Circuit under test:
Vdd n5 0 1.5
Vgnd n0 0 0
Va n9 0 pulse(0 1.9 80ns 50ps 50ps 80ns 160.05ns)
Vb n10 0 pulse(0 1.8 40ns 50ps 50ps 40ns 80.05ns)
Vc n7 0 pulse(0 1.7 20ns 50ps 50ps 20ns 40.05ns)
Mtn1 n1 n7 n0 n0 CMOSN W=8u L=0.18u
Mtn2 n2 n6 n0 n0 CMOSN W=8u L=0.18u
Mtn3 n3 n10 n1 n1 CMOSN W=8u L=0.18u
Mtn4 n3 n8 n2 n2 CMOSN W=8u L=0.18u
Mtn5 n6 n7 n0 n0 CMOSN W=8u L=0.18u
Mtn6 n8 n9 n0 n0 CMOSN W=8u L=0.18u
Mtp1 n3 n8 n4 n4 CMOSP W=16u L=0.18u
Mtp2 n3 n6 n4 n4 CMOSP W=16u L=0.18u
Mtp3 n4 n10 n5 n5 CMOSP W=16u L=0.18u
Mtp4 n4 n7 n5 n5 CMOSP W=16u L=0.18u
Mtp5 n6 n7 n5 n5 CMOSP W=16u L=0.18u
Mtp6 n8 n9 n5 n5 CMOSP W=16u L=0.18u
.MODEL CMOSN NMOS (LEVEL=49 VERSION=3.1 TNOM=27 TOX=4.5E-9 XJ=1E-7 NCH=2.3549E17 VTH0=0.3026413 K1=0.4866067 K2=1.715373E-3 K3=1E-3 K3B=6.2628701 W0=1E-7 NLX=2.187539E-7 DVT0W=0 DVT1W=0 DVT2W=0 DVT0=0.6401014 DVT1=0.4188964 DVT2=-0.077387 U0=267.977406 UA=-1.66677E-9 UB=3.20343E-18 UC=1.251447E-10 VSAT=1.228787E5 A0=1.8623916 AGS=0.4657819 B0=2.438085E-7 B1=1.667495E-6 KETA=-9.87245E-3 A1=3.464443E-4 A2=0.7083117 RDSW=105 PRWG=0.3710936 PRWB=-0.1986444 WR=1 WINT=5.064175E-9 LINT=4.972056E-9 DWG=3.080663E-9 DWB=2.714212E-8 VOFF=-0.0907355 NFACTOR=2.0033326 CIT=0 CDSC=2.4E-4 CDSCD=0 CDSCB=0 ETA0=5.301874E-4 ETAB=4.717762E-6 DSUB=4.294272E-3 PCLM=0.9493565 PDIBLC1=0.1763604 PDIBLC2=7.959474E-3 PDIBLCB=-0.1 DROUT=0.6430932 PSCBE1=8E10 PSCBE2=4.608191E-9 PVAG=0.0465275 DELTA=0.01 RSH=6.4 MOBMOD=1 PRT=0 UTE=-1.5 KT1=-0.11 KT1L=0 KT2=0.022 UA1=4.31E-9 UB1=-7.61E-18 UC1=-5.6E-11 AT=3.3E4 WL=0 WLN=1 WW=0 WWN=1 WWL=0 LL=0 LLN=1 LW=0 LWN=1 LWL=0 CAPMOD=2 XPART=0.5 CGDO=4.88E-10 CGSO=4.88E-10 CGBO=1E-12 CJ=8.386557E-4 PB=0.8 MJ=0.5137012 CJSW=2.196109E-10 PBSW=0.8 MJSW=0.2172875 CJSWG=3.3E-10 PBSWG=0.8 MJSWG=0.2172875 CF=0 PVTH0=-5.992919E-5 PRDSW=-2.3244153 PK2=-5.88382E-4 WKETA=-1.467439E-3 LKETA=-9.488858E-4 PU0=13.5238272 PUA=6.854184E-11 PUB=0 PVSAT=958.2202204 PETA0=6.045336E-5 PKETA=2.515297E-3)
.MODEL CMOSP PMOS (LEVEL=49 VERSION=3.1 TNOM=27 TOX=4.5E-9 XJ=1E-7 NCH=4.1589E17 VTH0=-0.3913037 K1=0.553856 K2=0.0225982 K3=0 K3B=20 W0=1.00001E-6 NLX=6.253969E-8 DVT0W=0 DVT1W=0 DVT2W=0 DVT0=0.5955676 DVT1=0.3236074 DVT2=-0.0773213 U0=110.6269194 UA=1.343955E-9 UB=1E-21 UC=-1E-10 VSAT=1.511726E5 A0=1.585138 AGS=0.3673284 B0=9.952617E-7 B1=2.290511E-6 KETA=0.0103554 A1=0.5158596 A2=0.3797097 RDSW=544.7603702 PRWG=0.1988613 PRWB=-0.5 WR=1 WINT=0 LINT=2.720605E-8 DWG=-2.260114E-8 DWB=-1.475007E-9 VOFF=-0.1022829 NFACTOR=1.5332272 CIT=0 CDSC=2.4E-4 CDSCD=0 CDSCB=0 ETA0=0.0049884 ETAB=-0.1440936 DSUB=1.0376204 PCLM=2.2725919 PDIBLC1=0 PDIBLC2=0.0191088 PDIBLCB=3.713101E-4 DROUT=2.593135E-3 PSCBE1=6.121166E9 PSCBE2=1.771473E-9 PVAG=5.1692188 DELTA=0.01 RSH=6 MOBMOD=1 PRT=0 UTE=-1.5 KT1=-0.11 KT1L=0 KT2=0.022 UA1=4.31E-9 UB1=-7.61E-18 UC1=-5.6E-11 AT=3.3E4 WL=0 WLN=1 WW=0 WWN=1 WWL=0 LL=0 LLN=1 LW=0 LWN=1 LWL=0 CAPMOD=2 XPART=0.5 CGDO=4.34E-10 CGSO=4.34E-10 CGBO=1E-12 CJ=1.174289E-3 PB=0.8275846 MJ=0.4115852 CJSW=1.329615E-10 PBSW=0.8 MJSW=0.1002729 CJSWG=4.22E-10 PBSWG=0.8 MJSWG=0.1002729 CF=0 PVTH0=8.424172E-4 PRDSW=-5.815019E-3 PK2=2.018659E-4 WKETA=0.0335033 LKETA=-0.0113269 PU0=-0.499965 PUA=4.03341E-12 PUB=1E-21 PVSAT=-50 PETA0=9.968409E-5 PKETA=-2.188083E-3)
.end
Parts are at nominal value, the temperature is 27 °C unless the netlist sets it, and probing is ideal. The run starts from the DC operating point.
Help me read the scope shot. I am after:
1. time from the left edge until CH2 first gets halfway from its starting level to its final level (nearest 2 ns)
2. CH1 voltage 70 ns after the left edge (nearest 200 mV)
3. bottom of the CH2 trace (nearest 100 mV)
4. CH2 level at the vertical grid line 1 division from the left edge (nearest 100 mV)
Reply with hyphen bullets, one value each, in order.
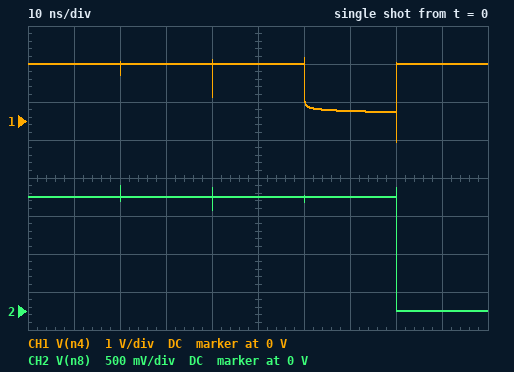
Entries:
- 80 ns
- 200 mV
- 0 V
- 1.5 V
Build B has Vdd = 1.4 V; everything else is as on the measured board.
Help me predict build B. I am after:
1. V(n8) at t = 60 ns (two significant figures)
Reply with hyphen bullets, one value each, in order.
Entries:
- 1.4 V
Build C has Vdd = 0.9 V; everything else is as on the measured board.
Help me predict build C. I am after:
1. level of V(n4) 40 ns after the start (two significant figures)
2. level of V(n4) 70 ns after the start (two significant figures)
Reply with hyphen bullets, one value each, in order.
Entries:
- 900 mV
- 250 mV
